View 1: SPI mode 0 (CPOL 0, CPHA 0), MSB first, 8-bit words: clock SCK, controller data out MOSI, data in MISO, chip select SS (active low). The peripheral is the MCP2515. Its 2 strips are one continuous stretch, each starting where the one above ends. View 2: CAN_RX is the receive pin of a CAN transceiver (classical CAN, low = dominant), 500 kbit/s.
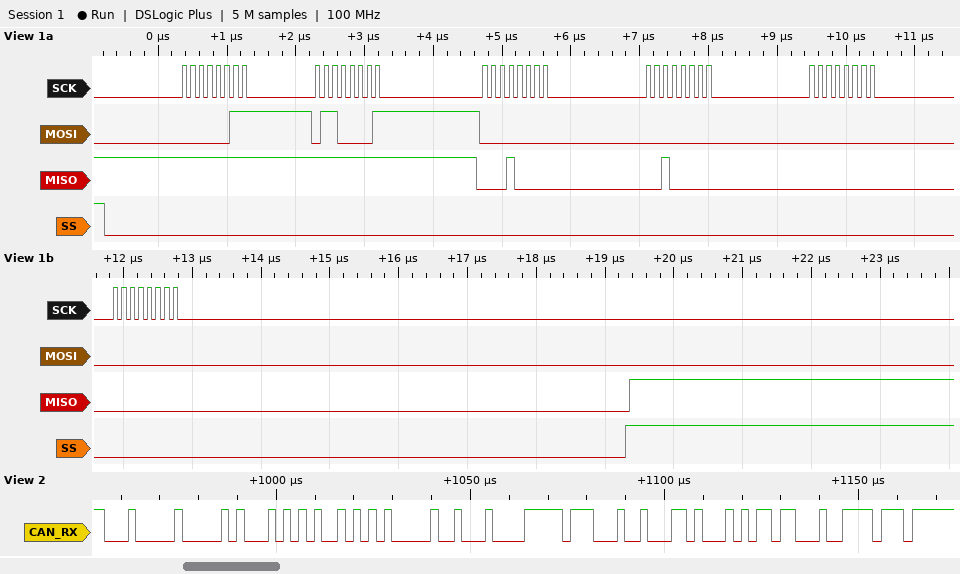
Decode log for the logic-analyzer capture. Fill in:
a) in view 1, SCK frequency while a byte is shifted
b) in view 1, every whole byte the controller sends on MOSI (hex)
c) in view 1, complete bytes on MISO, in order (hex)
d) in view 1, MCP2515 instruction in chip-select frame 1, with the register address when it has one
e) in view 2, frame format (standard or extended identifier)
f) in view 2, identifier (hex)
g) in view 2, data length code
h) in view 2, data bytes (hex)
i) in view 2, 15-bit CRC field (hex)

8 MHz
03 61 00 00 00 00
FF FF 10 20 00 00
READ 0x61
standard
0x100
8
AA 55 01 10 FF 12 34 56
0x627B
